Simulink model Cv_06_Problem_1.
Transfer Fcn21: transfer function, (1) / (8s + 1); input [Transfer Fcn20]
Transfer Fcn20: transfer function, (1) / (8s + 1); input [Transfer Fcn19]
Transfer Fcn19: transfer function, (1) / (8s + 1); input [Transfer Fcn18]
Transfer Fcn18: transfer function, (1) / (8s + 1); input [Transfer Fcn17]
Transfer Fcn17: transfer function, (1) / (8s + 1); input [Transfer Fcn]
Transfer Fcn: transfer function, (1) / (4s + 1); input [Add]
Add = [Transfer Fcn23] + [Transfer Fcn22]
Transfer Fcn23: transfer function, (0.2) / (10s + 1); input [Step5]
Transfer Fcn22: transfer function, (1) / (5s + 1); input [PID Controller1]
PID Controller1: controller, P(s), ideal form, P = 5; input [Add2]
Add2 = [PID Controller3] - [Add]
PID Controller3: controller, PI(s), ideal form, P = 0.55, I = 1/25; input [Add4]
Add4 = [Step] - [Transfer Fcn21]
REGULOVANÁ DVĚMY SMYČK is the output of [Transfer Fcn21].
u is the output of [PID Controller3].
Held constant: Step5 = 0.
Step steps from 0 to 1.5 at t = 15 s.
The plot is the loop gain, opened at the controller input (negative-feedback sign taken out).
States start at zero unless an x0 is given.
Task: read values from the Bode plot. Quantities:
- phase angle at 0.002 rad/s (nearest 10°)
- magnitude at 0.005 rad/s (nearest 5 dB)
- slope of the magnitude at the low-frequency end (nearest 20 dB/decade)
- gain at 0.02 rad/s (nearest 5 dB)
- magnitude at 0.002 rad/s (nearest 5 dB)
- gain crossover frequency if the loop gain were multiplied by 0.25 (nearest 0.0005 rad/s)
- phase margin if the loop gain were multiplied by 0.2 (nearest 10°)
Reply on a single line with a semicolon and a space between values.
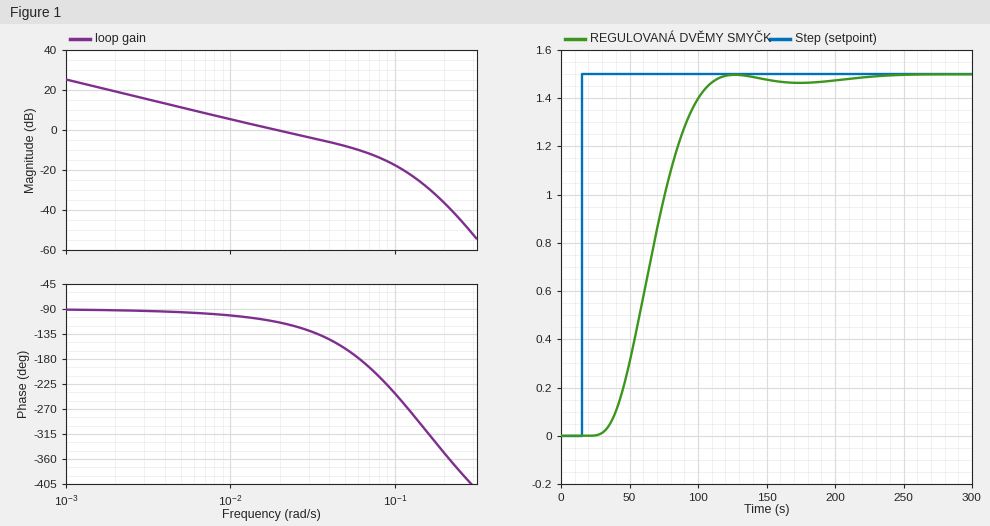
-90°; 10 dB; -20 dB/decade; 0 dB; 20 dB; 0.0045 rad/s; 90°
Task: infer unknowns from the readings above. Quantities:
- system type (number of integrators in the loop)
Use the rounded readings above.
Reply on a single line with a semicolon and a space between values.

1
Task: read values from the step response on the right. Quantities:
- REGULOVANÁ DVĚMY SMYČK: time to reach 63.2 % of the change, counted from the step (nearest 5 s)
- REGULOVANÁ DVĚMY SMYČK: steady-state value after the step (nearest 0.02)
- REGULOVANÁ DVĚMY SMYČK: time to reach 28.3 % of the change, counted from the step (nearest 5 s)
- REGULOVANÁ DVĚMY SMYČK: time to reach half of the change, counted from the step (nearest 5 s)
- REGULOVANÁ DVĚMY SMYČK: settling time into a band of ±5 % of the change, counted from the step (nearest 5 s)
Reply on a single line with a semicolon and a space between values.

60 s; 1.50; 40 s; 50 s; 90 s
